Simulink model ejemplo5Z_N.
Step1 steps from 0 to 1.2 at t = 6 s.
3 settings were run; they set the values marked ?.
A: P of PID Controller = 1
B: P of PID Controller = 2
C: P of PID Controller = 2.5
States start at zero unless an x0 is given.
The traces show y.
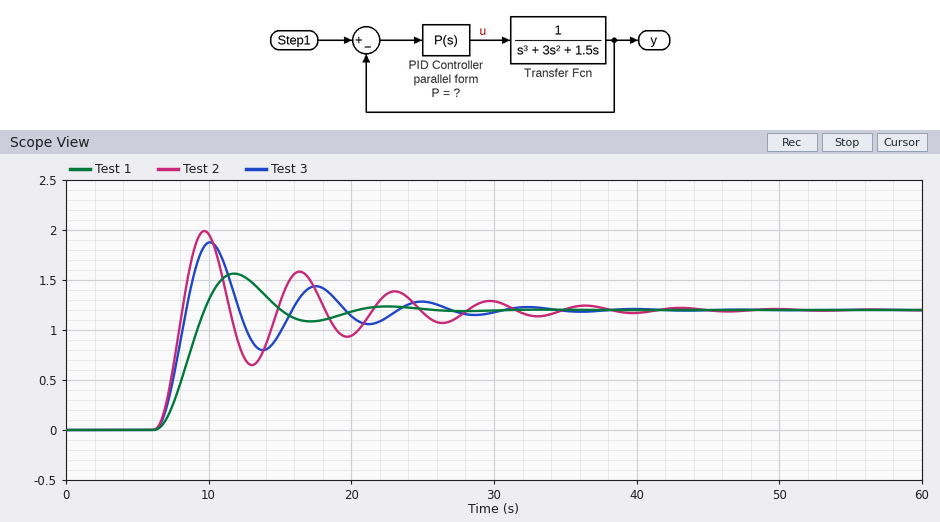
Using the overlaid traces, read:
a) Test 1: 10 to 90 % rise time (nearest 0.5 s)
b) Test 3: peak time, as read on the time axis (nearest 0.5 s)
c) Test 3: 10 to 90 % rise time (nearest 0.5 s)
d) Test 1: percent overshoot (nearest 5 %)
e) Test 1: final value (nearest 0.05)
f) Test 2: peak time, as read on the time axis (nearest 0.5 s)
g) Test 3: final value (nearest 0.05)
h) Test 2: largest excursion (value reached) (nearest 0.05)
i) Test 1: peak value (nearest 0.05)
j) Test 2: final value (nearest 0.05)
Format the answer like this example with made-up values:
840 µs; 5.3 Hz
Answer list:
2.5 s; 10.0 s; 1.5 s; 30 %; 1.20; 9.5 s; 1.20; 2.00; 1.55; 1.20
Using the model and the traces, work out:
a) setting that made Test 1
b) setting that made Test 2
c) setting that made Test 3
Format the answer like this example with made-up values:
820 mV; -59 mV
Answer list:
A; C; B
